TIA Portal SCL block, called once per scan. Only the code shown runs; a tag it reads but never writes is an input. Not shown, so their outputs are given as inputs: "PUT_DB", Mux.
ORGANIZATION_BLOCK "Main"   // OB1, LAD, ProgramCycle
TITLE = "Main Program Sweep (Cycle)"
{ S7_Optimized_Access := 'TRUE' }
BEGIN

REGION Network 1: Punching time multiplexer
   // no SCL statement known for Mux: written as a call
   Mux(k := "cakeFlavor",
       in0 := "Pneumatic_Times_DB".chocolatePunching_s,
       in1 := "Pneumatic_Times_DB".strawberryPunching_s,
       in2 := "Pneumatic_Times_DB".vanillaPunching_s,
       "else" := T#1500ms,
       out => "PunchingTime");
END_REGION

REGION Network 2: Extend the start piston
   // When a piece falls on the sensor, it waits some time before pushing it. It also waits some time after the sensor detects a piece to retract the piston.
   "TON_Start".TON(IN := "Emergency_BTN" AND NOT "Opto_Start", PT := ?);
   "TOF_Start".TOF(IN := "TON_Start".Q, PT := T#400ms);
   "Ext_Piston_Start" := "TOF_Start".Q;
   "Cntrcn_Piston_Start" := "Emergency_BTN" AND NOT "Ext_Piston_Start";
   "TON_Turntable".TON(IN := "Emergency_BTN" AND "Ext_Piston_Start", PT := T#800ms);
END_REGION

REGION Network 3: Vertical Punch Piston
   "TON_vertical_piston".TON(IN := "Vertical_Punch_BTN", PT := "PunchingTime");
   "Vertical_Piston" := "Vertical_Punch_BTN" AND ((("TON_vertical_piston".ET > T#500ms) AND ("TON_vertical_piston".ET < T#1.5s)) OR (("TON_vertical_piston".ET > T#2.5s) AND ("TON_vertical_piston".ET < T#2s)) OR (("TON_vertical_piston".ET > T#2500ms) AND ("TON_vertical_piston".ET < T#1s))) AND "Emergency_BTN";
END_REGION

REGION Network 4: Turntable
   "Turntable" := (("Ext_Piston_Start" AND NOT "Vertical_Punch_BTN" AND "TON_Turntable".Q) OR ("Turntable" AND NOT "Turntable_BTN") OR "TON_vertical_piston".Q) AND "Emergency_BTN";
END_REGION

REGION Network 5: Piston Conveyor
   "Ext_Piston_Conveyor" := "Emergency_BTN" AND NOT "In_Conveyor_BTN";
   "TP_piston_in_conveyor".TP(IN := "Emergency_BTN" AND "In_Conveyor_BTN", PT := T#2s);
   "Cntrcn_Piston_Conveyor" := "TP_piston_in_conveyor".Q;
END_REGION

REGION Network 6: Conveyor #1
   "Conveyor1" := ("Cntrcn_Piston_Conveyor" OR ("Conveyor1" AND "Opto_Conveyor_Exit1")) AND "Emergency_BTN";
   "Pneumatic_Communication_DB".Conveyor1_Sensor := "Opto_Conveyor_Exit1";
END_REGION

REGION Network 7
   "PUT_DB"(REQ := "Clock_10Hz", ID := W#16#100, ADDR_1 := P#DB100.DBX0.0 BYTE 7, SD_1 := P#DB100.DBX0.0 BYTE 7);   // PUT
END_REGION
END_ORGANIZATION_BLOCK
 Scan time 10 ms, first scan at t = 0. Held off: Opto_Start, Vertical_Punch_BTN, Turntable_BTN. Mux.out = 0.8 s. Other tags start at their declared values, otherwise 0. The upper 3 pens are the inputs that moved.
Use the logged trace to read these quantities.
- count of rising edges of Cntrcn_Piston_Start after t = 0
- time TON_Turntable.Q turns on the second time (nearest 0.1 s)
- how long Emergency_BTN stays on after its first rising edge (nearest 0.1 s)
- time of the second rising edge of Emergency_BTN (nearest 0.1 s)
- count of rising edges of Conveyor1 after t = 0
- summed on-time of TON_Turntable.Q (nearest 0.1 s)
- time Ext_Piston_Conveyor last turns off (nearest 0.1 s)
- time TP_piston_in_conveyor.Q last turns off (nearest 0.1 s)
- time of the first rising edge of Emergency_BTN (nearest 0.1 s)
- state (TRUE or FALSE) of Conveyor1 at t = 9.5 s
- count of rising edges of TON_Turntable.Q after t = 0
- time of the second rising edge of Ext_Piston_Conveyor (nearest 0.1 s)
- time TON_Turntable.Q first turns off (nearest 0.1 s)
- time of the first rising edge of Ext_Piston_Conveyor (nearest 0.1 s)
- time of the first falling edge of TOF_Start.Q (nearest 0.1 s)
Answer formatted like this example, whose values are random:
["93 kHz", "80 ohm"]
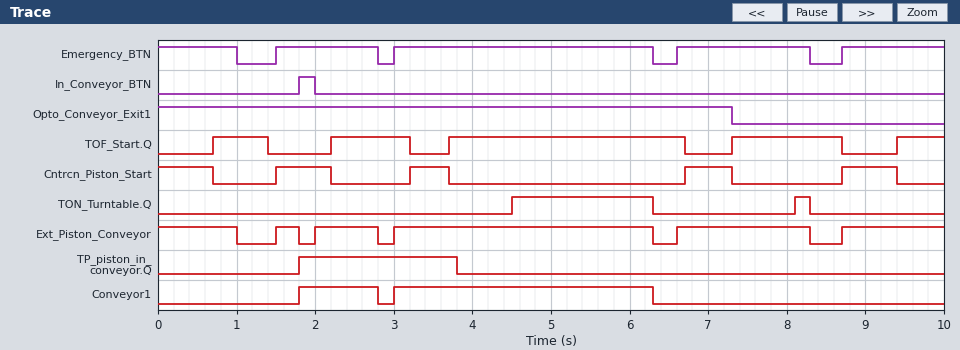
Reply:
["4", "8.1 s", "1.3 s", "3.0 s", "2", "2.0 s", "8.3 s", "3.8 s", "1.5 s", "FALSE", "2", "2.0 s", "6.3 s", "1.5 s", "1.4 s"]
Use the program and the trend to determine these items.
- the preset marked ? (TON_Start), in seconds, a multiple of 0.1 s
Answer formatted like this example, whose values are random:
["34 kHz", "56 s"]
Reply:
["0.7 s"]
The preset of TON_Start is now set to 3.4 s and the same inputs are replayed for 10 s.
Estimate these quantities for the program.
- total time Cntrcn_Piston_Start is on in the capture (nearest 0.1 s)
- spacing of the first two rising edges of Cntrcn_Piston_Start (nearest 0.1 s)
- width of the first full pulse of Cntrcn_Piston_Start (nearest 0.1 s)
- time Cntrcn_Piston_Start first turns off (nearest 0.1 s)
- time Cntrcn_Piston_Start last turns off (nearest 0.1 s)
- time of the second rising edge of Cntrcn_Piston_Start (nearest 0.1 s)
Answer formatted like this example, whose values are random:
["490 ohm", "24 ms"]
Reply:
["8.6 s", "1.5 s", "1.3 s", "1.0 s", "8.3 s", "3.0 s"]
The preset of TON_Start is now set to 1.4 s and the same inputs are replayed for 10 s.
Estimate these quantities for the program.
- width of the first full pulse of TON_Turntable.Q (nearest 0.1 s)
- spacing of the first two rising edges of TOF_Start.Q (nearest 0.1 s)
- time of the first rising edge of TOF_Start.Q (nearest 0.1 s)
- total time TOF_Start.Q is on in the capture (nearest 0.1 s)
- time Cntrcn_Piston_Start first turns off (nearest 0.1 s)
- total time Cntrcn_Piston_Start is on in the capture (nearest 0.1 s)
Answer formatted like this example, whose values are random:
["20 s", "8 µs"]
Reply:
["1.1 s", "3.6 s", "4.4 s", "3.0 s", "1.0 s", "6.3 s"]
